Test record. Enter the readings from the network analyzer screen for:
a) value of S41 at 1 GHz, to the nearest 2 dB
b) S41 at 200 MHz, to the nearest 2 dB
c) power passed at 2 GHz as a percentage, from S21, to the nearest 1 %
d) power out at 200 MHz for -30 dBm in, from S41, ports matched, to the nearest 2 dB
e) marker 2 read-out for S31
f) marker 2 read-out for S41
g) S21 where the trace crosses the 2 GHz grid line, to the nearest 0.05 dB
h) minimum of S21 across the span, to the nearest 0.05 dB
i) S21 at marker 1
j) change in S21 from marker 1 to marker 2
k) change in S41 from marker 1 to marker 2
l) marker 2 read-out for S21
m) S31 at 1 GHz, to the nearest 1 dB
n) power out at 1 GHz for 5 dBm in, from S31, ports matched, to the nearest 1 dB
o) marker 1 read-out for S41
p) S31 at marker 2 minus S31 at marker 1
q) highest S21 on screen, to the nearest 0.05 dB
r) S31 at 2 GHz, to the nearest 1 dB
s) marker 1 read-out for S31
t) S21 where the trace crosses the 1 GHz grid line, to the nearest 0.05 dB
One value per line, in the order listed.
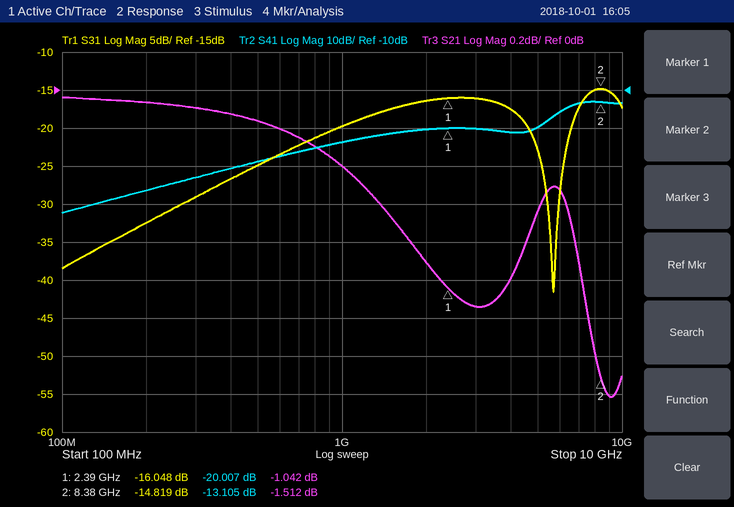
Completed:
-24 dB
-36 dB
81 %
-66 dBm
-14.819 dB
-13.105 dB
-0.90 dB
-1.60 dB
-1.042 dB
-0.470 dB
6.902 dB
-1.512 dB
-20 dB
-15 dBm
-20.007 dB
1.229 dB
-0.05 dB
-16 dB
-16.048 dB
-0.40 dB
